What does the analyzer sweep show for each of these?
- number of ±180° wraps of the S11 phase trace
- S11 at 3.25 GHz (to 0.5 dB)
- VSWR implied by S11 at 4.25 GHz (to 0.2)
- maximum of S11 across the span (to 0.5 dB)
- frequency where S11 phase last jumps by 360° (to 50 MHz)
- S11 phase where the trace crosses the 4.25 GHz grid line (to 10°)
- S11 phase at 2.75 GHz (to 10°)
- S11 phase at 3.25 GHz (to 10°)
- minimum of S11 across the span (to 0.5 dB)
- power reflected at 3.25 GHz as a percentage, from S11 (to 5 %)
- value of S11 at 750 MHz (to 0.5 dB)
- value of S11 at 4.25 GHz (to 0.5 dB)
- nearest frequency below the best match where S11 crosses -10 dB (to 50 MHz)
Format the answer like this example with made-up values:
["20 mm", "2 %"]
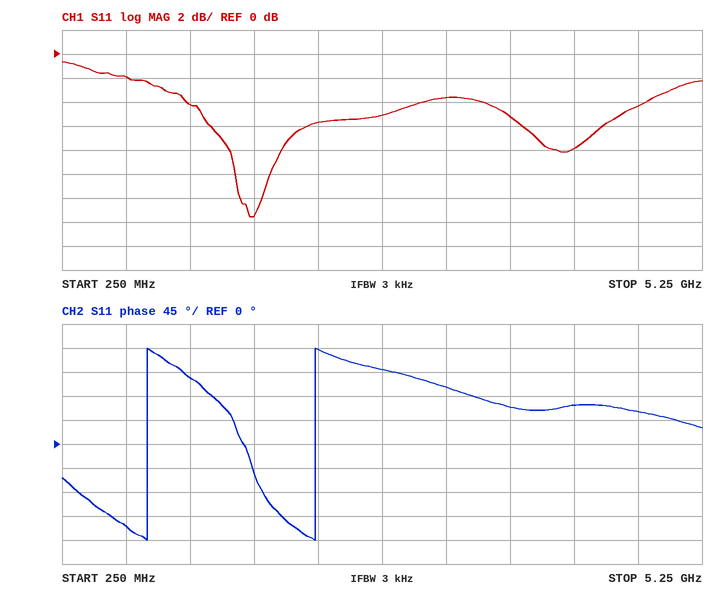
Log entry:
["2", "-3.5 dB", "2.4", "-0.5 dB", "2.25 GHz", "70°", "140°", "110°", "-13.5 dB", "45 %", "-2.0 dB", "-8.0 dB", "1.60 GHz"]
